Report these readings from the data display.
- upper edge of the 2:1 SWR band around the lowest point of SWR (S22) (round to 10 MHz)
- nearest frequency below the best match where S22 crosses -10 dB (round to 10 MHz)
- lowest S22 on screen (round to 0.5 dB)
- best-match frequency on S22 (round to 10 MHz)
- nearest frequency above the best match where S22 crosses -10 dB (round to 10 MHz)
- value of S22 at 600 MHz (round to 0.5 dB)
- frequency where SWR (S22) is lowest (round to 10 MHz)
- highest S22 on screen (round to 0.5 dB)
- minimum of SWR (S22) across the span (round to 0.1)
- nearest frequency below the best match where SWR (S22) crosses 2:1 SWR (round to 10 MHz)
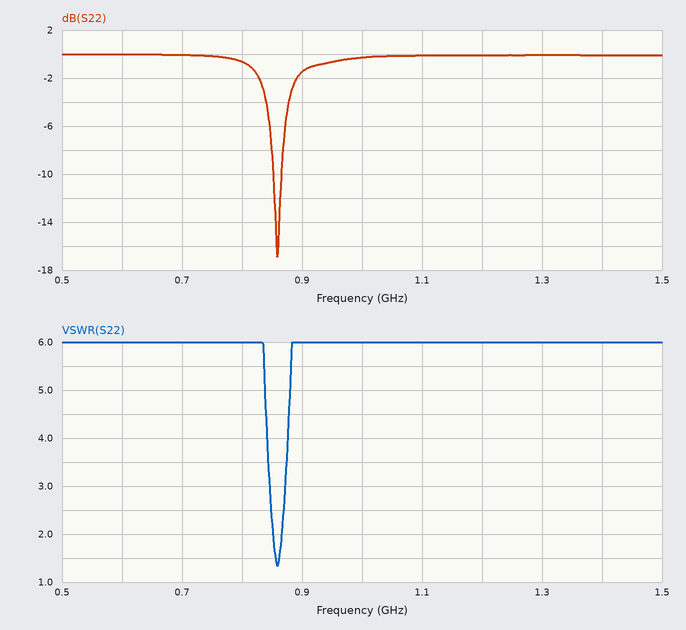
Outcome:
870 MHz
850 MHz
-17.0 dB
860 MHz
870 MHz
0.0 dB
860 MHz
0.0 dB
1.3
850 MHz
